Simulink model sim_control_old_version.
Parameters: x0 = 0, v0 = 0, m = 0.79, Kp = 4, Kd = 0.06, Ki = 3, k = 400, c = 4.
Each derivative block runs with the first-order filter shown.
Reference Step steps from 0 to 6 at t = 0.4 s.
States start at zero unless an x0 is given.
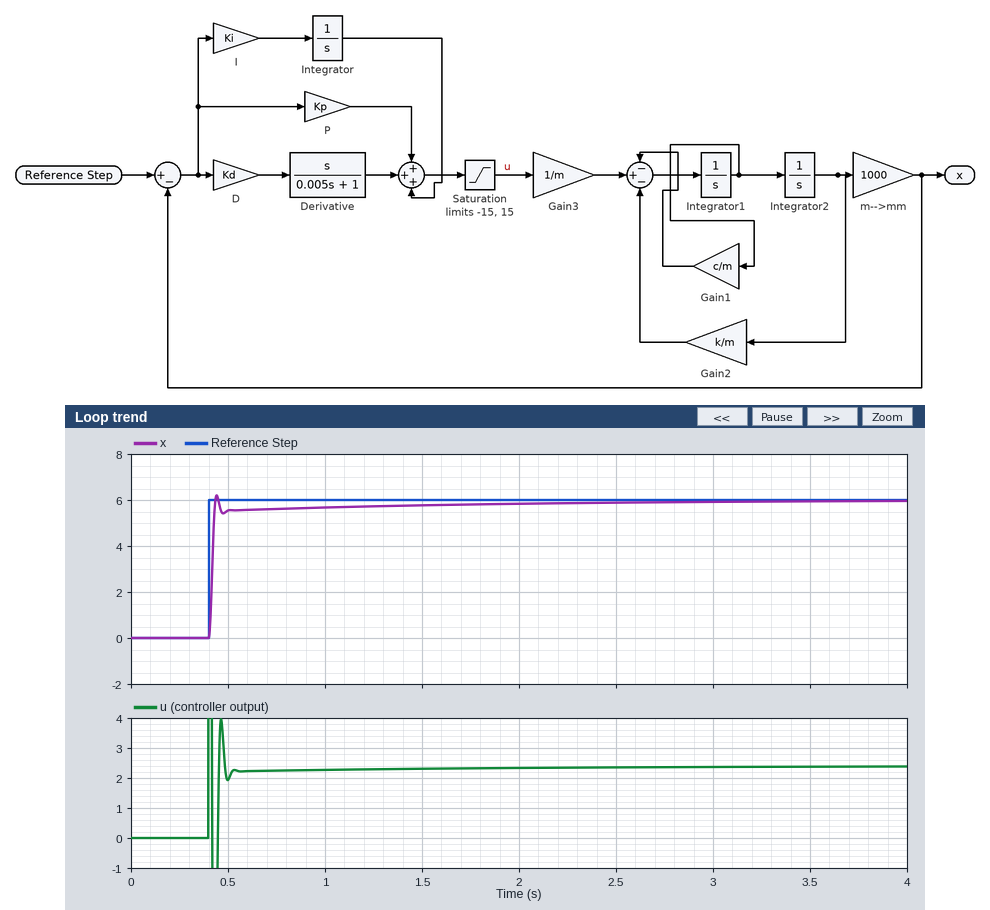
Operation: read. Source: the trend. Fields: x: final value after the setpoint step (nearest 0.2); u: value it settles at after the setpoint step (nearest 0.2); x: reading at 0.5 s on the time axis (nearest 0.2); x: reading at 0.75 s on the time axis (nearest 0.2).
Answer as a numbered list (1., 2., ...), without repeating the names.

1. 6.0
2. 2.4
3. 5.6
4. 5.6
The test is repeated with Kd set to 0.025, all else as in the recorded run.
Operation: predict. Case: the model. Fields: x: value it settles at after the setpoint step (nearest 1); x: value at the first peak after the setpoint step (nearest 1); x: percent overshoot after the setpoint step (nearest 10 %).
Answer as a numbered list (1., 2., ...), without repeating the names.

1. 6
2. 8
3. 30 %
